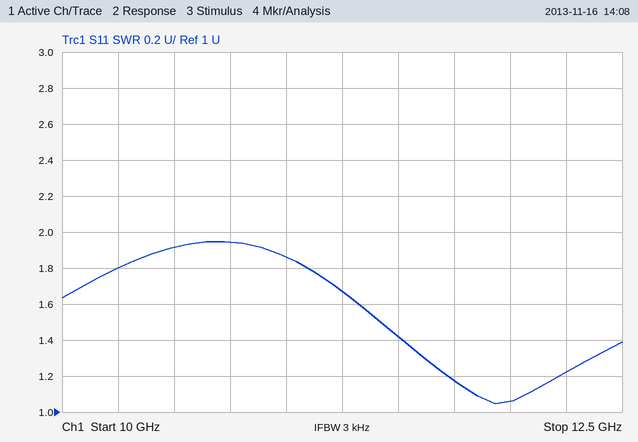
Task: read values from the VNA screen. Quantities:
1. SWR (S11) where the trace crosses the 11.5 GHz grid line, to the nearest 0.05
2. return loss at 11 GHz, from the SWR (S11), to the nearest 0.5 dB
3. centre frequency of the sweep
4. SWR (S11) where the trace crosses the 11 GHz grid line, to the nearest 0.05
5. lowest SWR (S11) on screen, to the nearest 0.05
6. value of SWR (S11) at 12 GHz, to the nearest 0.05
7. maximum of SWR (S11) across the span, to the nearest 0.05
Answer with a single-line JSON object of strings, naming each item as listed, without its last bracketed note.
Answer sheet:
{"SWR (S11) where the trace crosses the 11.5 GHz grid line, to the nearest 0.05": "1.40", "return loss at 11 GHz, from the SWR (S11), to the nearest 0.5 dB": "10.5 dB", "centre frequency of the sweep": "11.25 GHz", "SWR (S11) where the trace crosses the 11 GHz grid line, to the nearest 0.05": "1.85", "lowest SWR (S11) on screen, to the nearest 0.05": "1.05", "value of SWR (S11) at 12 GHz, to the nearest 0.05": "1.05", "maximum of SWR (S11) across the span, to the nearest 0.05": "1.95"}
